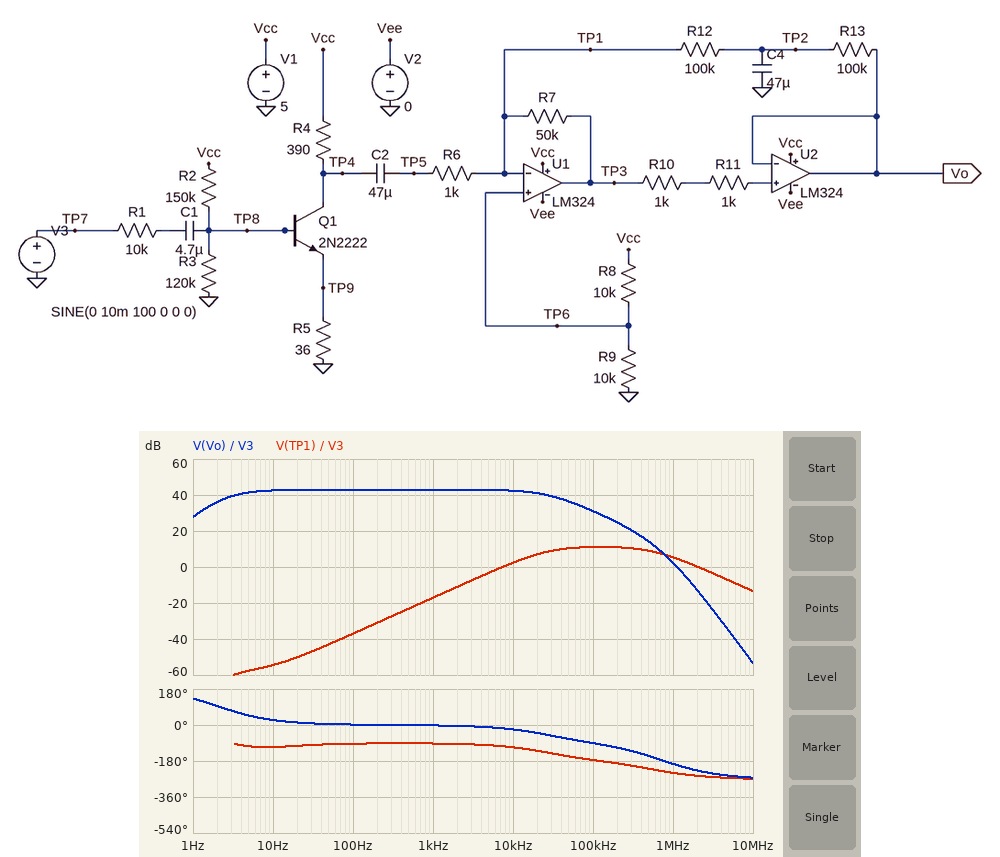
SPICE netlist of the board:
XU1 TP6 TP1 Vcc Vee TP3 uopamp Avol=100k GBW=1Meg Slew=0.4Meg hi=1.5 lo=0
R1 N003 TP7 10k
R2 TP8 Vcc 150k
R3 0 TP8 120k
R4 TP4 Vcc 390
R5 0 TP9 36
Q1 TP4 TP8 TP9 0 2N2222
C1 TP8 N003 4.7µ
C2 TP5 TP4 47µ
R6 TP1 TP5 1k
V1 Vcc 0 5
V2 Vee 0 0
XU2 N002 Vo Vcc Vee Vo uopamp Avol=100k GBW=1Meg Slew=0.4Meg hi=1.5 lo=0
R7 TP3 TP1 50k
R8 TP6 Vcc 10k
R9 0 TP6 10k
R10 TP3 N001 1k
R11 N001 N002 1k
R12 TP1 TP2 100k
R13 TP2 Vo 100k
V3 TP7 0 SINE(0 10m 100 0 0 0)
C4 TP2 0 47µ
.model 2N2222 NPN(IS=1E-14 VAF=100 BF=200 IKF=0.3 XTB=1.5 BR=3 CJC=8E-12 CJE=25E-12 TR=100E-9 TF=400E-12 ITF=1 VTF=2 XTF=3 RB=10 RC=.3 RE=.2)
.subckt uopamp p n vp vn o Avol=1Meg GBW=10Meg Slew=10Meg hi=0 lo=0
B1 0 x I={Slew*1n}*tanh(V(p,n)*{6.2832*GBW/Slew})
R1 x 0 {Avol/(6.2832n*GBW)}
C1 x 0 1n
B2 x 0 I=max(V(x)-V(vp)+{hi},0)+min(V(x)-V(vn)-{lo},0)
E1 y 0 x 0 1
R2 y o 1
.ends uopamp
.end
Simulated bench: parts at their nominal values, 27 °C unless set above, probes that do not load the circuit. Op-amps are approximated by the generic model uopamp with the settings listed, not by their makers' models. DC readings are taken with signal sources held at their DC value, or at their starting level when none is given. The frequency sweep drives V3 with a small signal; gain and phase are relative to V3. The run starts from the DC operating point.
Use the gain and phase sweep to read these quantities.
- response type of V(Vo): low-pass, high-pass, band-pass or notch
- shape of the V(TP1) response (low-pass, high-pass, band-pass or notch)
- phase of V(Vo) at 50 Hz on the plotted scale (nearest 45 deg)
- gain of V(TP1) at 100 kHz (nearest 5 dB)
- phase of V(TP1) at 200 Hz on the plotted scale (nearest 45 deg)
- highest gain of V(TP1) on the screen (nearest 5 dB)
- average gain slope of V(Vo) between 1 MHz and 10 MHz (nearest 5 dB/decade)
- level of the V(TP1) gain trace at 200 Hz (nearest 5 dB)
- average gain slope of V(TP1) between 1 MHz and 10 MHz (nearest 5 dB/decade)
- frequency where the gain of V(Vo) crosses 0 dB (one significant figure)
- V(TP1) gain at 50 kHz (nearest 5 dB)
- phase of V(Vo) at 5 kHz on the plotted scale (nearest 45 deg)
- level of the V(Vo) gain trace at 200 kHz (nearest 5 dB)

band-pass
band-pass
0 deg
10 dB
-90 deg
10 dB
-55 dB/decade
-30 dB
-20 dB/decade
1 MHz
10 dB
0 deg
25 dB
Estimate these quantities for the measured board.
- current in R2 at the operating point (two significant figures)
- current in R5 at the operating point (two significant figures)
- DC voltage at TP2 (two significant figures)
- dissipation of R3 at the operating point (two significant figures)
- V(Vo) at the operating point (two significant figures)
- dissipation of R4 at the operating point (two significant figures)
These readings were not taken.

28 µA
4.2 mA
2.5 V
5.9 µW
2.5 V
6.8 mW
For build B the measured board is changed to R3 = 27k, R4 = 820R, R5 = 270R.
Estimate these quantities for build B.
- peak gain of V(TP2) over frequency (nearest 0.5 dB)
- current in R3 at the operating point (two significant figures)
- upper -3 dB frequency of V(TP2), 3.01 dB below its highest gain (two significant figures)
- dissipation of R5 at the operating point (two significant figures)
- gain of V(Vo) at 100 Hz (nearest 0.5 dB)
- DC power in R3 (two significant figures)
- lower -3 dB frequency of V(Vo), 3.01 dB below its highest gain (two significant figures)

-7.0 dB
27 µA
3.7 Hz
34 µW
32.5 dB
19 µW
2.4 Hz
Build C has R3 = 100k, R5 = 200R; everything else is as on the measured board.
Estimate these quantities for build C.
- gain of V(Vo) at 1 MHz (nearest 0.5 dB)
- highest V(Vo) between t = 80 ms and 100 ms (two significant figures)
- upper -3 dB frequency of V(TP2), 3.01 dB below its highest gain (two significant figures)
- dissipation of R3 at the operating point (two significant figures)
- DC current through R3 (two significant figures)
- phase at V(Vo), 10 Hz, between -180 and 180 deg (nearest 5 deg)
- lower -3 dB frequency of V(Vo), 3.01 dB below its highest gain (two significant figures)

-3.0 dB
3.0 V
4.0 Hz
15 µW
12 µA
20 deg
2.8 Hz
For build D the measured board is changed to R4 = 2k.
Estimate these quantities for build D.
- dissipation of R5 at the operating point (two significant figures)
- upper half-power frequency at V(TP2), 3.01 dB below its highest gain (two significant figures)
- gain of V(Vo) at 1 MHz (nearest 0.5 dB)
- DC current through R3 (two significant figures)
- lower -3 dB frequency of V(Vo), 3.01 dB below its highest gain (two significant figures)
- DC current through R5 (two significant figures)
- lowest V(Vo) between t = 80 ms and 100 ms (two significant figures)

210 µW
7.8 Hz
-22.5 dB
6.4 µA
5.0 Hz
2.4 mA
2.4 V
